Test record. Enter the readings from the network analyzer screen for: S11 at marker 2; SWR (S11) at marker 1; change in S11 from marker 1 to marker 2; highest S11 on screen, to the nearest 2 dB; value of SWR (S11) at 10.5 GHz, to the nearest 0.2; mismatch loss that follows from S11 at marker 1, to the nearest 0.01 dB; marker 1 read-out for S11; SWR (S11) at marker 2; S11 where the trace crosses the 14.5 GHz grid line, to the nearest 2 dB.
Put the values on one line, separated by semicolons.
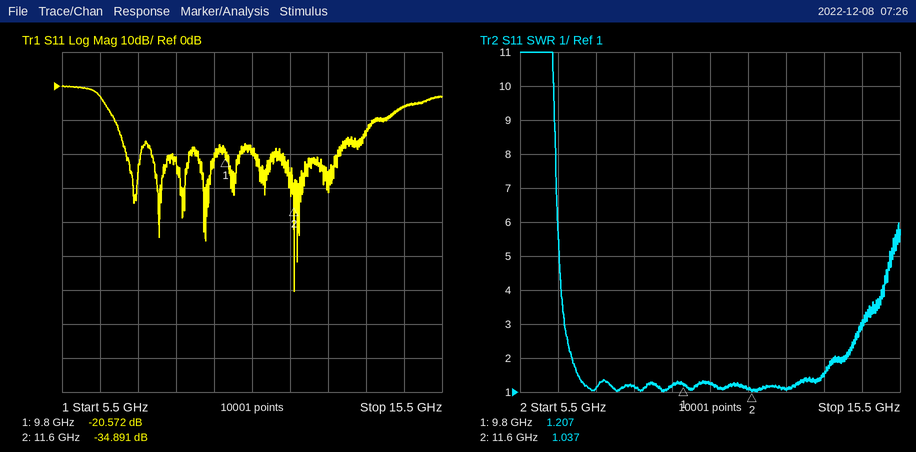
-34.891 dB; 1.207; -14.319 dB; 0 dB; 1.2; 0.04 dB; -20.572 dB; 1.037; -6 dB
